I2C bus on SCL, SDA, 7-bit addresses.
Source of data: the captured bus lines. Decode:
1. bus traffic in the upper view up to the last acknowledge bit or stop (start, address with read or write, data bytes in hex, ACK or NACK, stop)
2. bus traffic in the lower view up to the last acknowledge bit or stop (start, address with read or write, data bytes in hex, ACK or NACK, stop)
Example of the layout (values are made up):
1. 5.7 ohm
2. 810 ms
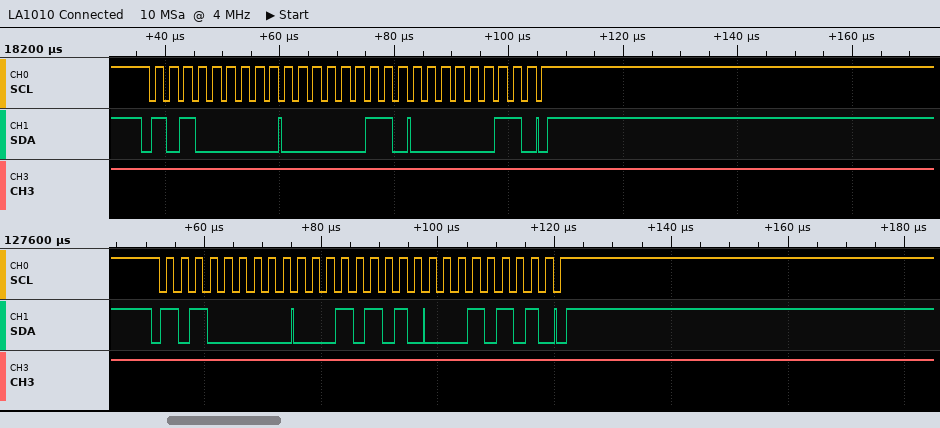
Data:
1. start, address 50 write ACK, 03 ACK, 03 ACK, stop
2. start, address 50 write ACK, 15 ACK, 15 ACK, stop
